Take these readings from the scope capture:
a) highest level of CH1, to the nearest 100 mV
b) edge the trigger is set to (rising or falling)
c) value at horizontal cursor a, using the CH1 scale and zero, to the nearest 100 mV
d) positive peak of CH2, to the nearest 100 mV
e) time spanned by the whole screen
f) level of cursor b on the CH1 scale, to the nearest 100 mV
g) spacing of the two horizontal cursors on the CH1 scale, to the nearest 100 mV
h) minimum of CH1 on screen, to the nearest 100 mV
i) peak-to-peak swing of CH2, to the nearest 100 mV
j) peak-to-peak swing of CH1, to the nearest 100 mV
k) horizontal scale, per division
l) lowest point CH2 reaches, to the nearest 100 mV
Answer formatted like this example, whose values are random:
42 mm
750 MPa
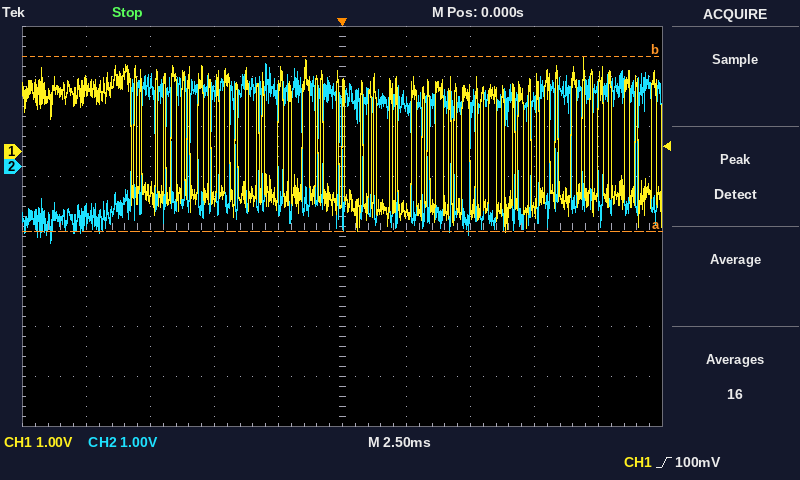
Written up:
1.9 V
rising
-1.6 V
2.1 V
25 ms
1.9 V
3.5 V
-1.6 V
3.6 V
3.5 V
2.5 ms
-1.5 V
